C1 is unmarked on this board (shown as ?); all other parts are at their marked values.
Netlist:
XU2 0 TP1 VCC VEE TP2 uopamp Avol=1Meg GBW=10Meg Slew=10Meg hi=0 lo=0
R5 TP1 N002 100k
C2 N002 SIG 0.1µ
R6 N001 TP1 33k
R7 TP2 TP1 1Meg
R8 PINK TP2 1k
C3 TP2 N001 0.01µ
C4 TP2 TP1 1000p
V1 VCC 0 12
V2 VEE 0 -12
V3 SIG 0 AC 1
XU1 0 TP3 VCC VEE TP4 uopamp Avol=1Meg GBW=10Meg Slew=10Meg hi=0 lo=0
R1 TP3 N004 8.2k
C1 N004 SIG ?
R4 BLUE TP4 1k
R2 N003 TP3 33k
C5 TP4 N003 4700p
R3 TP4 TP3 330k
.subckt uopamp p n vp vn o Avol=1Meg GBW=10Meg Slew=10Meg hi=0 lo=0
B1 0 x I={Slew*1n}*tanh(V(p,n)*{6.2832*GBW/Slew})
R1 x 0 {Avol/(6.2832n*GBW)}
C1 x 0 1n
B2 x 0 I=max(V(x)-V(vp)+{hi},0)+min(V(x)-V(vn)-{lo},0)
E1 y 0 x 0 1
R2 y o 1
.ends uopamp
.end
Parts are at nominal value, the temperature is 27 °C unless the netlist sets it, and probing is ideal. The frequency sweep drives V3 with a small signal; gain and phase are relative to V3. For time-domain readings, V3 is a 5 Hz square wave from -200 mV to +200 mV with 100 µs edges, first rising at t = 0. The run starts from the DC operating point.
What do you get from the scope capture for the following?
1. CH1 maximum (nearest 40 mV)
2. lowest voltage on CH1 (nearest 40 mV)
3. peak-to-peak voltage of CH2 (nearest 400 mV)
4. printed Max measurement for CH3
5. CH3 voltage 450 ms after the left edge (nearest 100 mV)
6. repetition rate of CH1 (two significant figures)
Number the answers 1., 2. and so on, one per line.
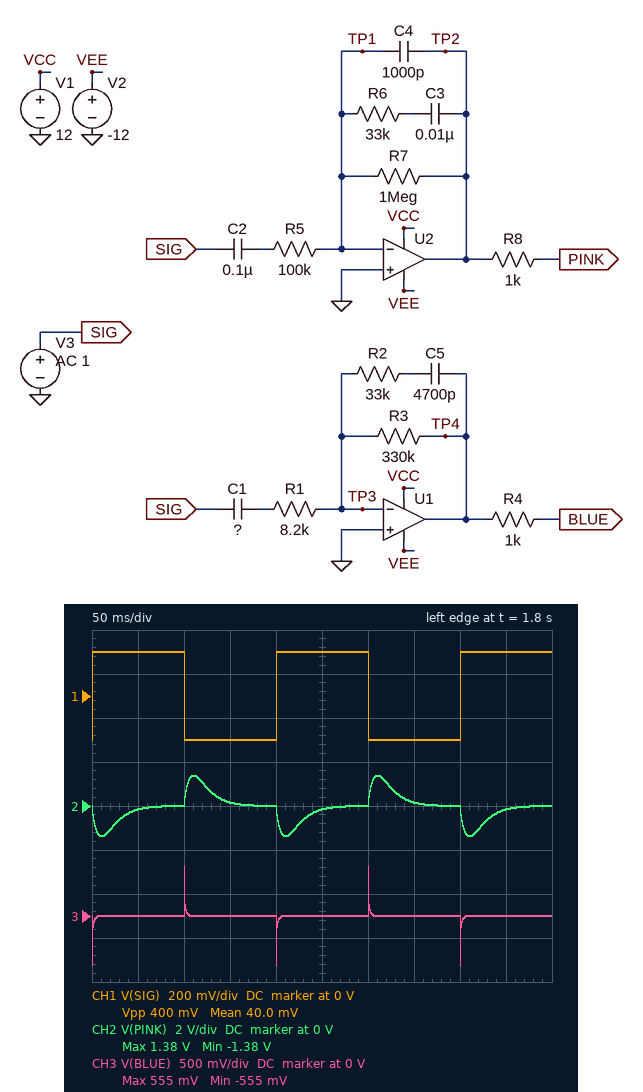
1. 200 mV
2. -200 mV
3. 2.8 V
4. 555 mV
5. 0 V
6. 5.0 Hz
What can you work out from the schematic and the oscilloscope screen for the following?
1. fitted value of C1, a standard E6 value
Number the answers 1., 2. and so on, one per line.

1. 3.3 nF
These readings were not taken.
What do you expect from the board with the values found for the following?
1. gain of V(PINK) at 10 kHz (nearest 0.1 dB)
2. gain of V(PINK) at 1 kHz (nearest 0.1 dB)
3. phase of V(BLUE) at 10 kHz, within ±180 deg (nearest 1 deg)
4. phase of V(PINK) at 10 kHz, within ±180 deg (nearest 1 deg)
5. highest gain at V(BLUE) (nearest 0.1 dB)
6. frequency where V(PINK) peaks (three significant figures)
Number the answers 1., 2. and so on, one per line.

1. -17.1 dB
2. -9.9 dB
3. -155 deg
4. 116 deg
5. 11.3 dB
6. 15.0 Hz
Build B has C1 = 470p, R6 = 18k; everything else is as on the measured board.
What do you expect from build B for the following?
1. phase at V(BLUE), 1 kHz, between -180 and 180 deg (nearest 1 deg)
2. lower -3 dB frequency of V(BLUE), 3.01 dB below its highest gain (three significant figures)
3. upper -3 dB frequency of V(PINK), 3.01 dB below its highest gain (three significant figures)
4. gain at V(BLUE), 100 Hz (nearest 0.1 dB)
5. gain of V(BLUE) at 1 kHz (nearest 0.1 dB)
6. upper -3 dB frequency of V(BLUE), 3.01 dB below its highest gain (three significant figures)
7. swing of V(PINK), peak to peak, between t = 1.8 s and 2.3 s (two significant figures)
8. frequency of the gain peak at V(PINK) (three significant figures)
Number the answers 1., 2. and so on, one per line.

1. -132 deg
2. 40.3 kHz
3. 36.4 Hz
4. -23.5 dB
5. -18.0 dB
6. 2.20 MHz
7. 2.8 V
8. 15.1 Hz
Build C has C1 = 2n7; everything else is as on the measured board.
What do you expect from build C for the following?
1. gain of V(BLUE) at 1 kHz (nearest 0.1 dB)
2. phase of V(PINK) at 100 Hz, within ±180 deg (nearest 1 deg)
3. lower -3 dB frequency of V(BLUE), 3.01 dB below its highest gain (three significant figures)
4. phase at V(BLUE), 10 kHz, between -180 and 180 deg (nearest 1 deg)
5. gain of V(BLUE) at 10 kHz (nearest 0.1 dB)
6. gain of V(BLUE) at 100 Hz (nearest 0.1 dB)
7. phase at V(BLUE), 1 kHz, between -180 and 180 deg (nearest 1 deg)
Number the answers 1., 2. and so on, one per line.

1. -2.9 dB
2. 118 deg
3. 7.01 kHz
4. -150 deg
5. 9.5 dB
6. -8.3 dB
7. -138 deg
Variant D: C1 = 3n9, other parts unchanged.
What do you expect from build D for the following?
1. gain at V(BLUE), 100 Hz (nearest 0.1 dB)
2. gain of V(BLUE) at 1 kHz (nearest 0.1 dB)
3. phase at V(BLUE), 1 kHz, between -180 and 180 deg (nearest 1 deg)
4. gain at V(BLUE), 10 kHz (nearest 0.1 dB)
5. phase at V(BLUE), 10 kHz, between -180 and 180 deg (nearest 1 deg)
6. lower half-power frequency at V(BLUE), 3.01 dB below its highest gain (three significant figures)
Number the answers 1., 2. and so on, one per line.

1. -5.1 dB
2. 0.2 dB
3. -142 deg
4. 10.4 dB
5. -159 deg
6. 4.75 kHz
